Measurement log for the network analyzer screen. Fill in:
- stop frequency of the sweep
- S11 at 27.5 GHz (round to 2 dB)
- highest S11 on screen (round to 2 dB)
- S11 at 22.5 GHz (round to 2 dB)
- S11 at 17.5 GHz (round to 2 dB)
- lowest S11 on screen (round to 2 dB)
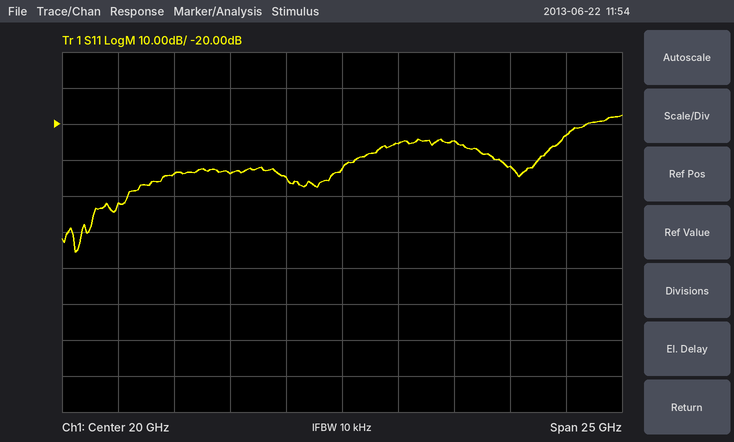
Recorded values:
32.5 GHz
-32 dB
-18 dB
-26 dB
-34 dB
-56 dB
